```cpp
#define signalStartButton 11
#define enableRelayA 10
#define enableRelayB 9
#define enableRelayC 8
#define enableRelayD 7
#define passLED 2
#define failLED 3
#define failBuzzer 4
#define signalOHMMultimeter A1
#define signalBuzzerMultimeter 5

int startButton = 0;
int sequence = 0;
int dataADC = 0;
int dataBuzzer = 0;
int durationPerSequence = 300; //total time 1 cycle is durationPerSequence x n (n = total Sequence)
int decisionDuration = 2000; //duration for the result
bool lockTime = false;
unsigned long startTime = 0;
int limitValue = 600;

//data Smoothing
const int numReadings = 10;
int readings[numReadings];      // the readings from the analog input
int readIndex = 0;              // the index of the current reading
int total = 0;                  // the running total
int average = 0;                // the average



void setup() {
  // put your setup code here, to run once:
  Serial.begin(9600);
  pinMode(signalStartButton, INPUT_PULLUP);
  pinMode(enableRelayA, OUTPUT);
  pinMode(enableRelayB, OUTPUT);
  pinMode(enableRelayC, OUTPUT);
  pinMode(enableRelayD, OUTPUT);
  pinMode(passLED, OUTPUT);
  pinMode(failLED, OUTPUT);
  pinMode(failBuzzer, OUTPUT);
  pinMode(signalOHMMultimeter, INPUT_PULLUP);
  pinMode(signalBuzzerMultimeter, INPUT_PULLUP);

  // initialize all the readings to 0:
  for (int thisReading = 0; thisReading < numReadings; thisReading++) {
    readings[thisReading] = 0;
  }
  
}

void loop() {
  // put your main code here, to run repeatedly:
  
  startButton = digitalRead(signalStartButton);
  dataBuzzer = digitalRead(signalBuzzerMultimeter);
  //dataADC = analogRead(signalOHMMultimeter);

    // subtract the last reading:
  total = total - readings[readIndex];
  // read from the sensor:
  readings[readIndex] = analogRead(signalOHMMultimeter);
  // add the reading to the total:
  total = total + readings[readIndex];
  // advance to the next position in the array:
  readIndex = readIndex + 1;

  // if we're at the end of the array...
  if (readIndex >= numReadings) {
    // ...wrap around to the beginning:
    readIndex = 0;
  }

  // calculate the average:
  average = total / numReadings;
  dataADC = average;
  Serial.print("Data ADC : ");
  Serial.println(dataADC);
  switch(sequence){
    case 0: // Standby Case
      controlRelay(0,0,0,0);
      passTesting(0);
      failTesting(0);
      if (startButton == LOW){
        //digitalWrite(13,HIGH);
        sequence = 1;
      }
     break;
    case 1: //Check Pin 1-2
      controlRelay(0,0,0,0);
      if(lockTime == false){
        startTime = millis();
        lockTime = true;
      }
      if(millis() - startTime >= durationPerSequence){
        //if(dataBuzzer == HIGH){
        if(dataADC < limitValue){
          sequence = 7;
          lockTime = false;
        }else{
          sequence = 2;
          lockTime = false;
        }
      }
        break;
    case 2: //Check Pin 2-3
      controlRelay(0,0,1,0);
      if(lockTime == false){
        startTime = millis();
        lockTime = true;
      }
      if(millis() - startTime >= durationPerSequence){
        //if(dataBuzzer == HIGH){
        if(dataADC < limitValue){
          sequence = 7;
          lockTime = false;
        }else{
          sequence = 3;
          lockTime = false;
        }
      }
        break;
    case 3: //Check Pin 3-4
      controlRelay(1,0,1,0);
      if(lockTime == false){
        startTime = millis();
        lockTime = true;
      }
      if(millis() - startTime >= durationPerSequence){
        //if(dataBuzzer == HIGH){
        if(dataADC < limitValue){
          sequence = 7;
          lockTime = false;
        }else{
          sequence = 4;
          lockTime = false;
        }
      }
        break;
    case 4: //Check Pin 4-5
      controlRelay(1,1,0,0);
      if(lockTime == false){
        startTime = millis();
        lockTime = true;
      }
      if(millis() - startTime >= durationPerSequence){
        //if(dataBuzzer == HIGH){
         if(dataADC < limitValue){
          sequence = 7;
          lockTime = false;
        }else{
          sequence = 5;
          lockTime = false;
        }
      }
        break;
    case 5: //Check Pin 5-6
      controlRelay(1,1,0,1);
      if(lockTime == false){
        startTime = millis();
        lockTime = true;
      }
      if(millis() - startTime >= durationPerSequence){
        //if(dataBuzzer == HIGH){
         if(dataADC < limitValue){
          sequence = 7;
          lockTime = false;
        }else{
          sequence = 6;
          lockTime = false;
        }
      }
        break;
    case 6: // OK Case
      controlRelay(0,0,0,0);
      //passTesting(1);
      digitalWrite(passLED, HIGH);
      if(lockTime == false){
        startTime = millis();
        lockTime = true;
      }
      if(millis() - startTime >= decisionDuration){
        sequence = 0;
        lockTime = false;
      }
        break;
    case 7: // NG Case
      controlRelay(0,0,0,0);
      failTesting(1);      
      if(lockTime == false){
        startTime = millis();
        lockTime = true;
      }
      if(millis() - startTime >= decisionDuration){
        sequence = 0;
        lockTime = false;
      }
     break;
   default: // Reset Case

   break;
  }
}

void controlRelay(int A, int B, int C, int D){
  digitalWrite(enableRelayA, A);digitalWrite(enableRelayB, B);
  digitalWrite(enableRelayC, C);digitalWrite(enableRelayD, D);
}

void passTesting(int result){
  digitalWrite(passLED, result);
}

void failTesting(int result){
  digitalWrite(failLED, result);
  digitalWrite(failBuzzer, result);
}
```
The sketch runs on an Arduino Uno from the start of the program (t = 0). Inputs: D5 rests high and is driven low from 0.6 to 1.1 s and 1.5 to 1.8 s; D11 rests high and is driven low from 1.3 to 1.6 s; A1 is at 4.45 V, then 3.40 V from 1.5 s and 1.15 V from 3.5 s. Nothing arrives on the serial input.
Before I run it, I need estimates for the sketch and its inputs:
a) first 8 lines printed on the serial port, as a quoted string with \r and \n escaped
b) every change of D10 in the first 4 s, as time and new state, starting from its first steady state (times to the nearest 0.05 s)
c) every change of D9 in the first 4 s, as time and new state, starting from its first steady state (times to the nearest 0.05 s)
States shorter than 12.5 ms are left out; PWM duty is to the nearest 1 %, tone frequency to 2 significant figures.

"Data ADC : 91\r\nData ADC : 182\r\nData ADC : 273\r\nData ADC : 364\r\nData ADC : 455\r\nData ADC : 546\r\nData ADC : 637\r\nData ADC : 728\r\n"
0 s low; 2 s high; 3 s low
0 s low; 2.35 s high; 3 s low
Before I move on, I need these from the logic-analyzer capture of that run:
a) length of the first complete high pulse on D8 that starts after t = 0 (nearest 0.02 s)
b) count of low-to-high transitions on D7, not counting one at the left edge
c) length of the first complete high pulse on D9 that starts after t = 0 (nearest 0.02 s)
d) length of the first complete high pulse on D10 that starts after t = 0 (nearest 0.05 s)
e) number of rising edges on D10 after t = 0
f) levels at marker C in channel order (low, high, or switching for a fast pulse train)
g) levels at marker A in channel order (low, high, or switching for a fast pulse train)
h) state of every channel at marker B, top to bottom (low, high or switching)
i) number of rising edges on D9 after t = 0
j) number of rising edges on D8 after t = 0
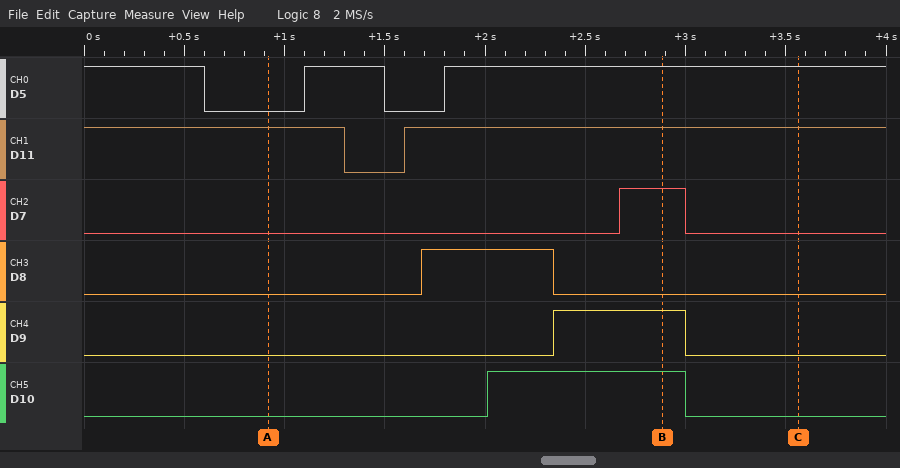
0.66 s
1
0.66 s
1.00 s
1
D5 high, D11 high, D7 low, D8 low, D9 low, D10 low
D5 low, D11 high, D7 low, D8 low, D9 low, D10 low
D5 high, D11 high, D7 high, D8 low, D9 high, D10 high
1
1
